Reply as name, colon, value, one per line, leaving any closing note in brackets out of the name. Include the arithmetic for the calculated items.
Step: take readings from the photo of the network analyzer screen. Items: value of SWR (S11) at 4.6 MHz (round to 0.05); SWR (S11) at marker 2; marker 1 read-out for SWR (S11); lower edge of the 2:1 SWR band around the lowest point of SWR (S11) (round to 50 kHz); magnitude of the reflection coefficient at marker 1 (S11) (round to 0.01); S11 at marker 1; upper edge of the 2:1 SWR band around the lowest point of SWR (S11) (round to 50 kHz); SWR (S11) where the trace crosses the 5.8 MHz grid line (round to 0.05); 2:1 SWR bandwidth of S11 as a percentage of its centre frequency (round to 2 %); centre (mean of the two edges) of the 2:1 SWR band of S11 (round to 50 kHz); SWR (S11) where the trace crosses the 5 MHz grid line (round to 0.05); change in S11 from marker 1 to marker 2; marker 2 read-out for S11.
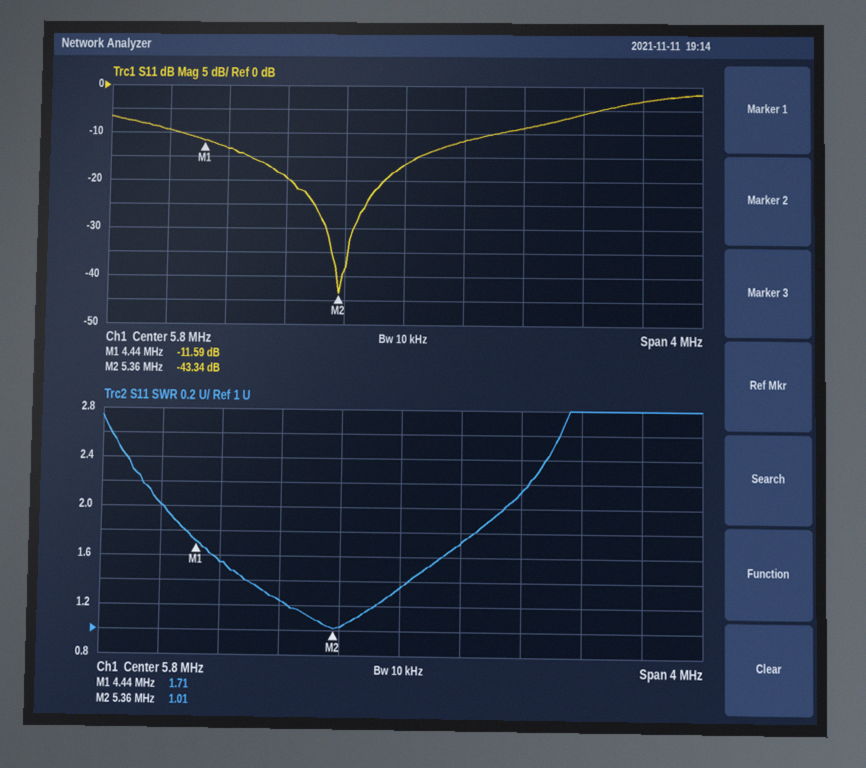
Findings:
value of SWR (S11) at 4.6 MHz: 1.55
SWR (S11) at marker 2: 1.01
marker 1 read-out for SWR: 1.71
lower edge of the 2:1 SWR band around the lowest point of SWR (S11): 4.20 MHz
magnitude of the reflection coefficient at marker 1 (S11): 10^(-11.59/20) ≈ 0.26
S11 at marker 1: -11.59 dB
upper edge of the 2:1 SWR band around the lowest point of SWR (S11): 6.50 MHz
SWR (S11) where the trace crosses the 5.8 MHz grid line: 1.35
2:1 SWR bandwidth of S11 as a percentage of its centre frequency: 2.3 MHz / 5.35 MHz ≈ 43.0 %, so 42 % to the nearest 2 %
centre (mean of the two edges) of the 2:1 SWR band of S11: 5.35 MHz
SWR (S11) where the trace crosses the 5 MHz grid line: 1.25
change in S11 from marker 1 to marker 2: -43.34 − (-11.59) = -31.75 dB
marker 2 read-out for S11: -43.34 dB
